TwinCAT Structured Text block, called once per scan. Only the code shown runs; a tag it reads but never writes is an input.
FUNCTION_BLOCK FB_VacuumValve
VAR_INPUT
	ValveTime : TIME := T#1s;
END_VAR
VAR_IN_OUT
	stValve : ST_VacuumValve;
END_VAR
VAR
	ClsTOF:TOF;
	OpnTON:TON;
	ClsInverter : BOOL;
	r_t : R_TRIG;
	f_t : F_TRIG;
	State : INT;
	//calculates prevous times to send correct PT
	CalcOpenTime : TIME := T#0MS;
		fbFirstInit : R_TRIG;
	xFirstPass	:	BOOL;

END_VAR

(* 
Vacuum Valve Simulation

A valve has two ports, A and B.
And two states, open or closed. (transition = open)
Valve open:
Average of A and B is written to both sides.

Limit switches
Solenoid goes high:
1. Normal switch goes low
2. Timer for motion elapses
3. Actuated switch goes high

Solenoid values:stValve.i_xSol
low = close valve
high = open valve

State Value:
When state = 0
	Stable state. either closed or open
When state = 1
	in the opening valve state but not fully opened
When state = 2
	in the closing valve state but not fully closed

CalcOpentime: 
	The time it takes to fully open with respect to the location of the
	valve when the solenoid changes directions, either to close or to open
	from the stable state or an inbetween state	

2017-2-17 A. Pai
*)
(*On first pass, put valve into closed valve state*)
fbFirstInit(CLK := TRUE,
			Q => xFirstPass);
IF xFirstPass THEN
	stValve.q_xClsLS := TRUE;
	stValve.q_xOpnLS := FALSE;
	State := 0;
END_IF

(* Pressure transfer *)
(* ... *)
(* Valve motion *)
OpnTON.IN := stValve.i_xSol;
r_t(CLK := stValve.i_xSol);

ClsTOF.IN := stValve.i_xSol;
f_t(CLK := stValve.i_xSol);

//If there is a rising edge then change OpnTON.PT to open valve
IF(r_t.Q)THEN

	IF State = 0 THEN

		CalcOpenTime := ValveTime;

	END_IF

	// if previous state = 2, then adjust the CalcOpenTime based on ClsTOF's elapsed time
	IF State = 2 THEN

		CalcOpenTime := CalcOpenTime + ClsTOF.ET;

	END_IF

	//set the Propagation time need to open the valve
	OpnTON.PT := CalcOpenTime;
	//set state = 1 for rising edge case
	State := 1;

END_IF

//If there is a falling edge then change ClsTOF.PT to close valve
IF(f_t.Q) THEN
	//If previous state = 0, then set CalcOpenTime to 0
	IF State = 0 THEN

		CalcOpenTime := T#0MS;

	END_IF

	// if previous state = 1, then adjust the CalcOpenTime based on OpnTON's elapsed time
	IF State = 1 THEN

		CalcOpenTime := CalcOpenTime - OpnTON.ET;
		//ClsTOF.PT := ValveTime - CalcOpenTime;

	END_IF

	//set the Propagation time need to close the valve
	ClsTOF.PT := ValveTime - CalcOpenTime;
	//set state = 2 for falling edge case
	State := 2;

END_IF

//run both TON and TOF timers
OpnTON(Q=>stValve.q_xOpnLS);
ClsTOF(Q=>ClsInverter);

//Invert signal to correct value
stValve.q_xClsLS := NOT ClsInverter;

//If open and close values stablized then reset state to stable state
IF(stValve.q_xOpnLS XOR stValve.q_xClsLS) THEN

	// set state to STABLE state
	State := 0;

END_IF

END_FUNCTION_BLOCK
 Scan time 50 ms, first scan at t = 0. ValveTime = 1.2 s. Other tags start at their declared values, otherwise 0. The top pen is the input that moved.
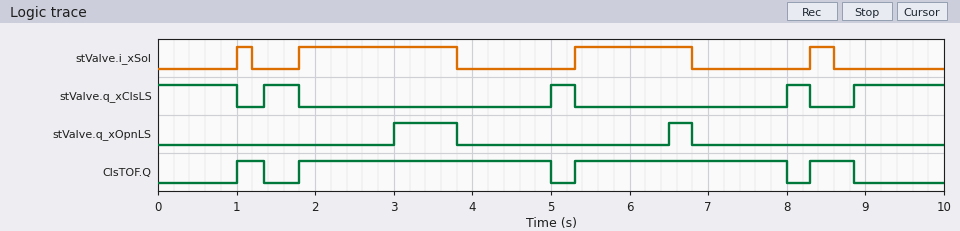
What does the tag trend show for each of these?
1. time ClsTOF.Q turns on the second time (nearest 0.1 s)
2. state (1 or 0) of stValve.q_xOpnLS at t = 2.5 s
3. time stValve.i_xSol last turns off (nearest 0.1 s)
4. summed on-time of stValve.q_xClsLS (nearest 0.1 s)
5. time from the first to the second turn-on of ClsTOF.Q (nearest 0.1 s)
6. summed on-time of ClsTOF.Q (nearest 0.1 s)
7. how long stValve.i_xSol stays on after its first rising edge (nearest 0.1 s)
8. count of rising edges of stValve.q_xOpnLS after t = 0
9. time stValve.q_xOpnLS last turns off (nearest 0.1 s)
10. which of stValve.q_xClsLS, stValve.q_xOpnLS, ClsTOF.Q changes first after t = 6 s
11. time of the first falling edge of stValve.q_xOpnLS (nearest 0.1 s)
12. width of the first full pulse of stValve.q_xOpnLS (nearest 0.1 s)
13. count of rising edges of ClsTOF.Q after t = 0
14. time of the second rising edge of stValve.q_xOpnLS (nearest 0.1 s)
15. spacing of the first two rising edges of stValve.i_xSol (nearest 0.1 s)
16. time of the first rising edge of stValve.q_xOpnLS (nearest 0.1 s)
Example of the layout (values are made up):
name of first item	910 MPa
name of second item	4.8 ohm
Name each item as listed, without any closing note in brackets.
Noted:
time ClsTOF.Q turns on the second time	1.8 s
state (1 or 0) of stValve.q_xOpnLS at t = 2.5 s	0
time stValve.i_xSol last turns off	8.6 s
summed on-time of stValve.q_xClsLS	3.2 s
time from the first to the second turn-on of ClsTOF.Q	0.8 s
summed on-time of ClsTOF.Q	6.8 s
how long stValve.i_xSol stays on after its first rising edge	0.2 s
count of rising edges of stValve.q_xOpnLS after t = 0	2
time stValve.q_xOpnLS last turns off	6.8 s
which of stValve.q_xClsLS, stValve.q_xOpnLS, ClsTOF.Q changes first after t = 6 s	stValve.q_xOpnLS
time of the first falling edge of stValve.q_xOpnLS	3.8 s
width of the first full pulse of stValve.q_xOpnLS	0.8 s
count of rising edges of ClsTOF.Q after t = 0	4
time of the second rising edge of stValve.q_xOpnLS	6.5 s
spacing of the first two rising edges of stValve.i_xSol	0.8 s
time of the first rising edge of stValve.q_xOpnLS	3.0 s
